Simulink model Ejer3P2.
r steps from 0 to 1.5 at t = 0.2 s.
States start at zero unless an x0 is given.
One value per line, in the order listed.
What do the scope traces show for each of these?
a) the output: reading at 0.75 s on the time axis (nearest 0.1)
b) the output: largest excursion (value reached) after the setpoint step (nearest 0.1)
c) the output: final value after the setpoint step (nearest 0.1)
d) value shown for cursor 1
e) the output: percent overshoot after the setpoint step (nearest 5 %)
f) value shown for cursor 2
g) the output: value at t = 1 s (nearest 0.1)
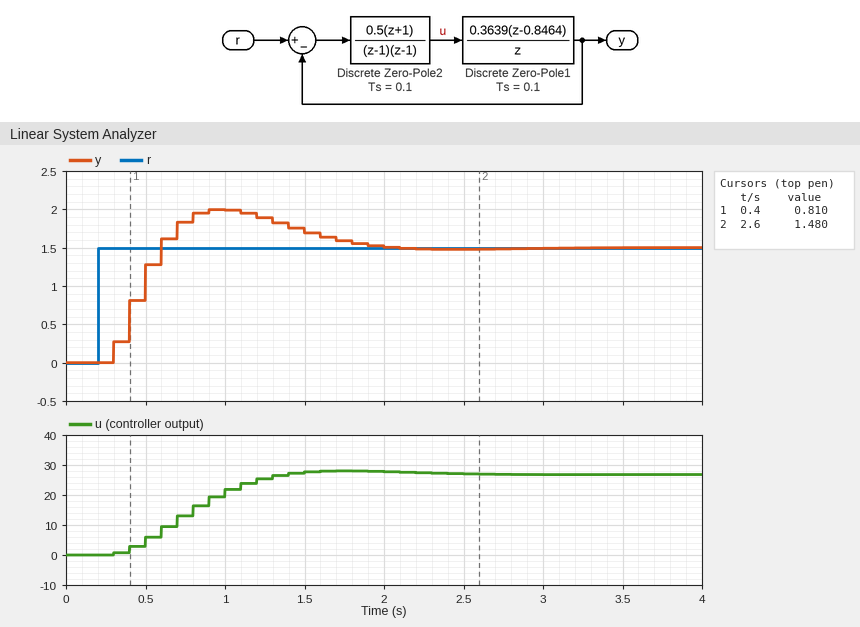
1.8
2.0
1.5
0.810
35 %
1.480
2.0
